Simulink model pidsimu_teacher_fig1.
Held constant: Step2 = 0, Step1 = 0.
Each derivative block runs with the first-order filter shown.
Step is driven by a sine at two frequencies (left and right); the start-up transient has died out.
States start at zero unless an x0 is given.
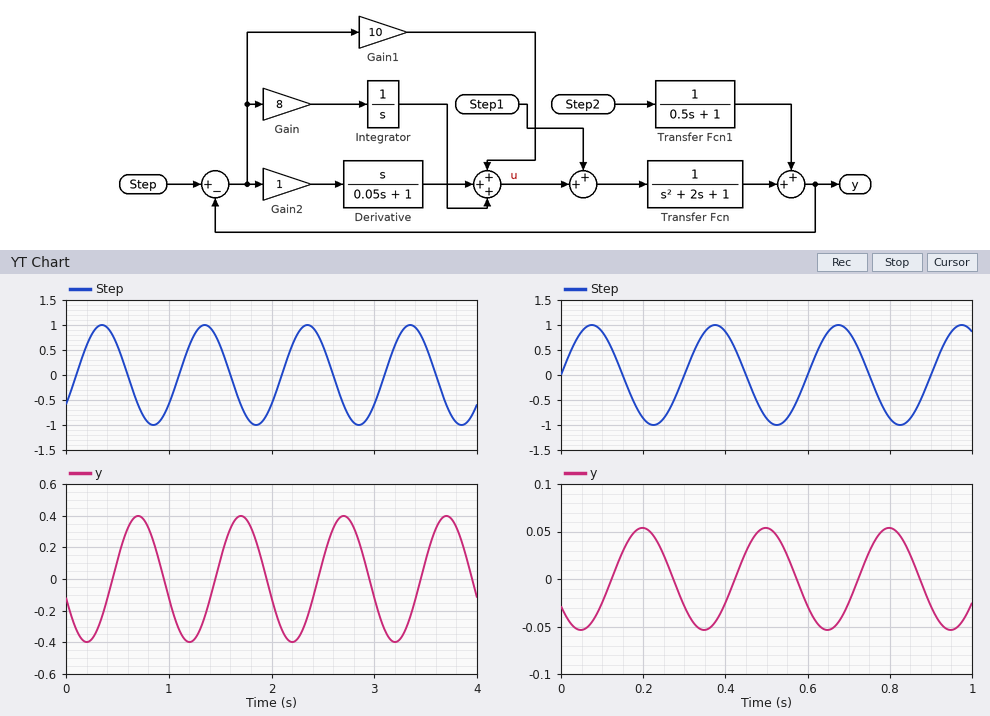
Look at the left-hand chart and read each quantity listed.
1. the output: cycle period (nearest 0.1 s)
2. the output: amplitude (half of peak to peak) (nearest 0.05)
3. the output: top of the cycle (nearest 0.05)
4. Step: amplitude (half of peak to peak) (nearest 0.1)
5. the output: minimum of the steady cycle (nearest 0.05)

1.0 s
0.40
0.40
1.0
-0.40
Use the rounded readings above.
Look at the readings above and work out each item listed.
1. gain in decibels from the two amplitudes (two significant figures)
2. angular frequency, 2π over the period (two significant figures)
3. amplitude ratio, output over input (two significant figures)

-8.0 dB
6.3 rad/s
0.40
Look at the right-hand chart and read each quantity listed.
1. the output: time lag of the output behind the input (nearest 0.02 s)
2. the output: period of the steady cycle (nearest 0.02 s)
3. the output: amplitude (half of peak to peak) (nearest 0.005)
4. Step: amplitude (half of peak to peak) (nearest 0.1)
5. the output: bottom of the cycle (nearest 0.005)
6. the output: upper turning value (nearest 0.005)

0.12 s
0.30 s
0.055
1.0
-0.055
0.055
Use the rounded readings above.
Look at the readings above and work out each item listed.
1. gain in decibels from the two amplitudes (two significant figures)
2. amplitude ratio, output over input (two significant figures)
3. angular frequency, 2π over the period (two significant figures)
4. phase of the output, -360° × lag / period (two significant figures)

-25 dB
0.055
21 rad/s
-140°
